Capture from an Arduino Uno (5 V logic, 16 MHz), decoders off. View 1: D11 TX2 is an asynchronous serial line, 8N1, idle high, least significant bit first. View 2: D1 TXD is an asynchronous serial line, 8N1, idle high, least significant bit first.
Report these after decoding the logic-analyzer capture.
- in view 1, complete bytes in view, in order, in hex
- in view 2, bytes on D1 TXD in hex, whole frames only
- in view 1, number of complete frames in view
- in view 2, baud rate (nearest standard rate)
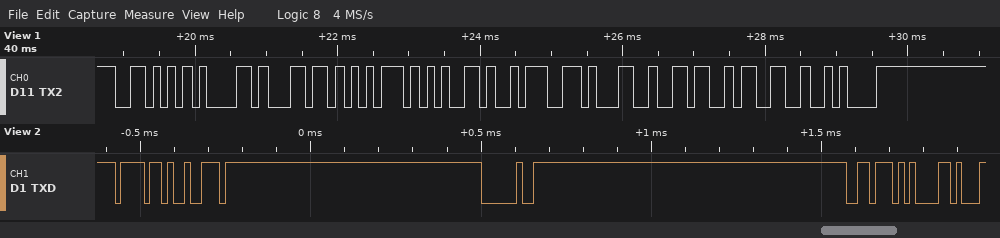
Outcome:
56 61 6C 75 65 3A 31 36 33 0A
6F 72 20 76 61
10
57600 baud
